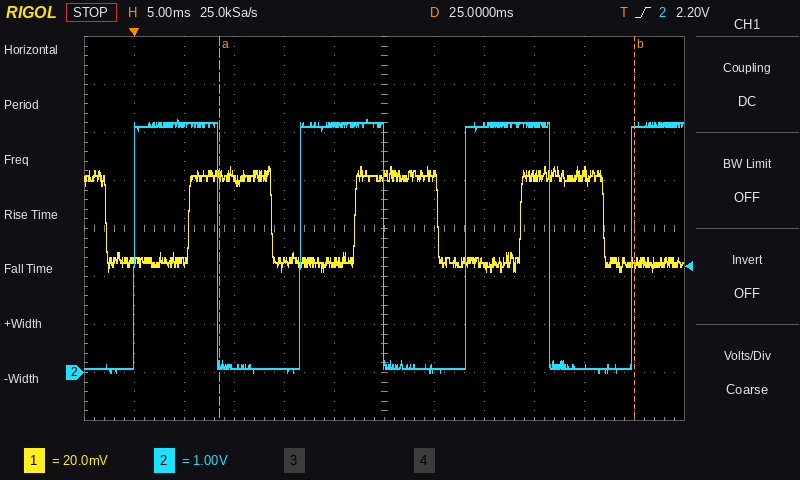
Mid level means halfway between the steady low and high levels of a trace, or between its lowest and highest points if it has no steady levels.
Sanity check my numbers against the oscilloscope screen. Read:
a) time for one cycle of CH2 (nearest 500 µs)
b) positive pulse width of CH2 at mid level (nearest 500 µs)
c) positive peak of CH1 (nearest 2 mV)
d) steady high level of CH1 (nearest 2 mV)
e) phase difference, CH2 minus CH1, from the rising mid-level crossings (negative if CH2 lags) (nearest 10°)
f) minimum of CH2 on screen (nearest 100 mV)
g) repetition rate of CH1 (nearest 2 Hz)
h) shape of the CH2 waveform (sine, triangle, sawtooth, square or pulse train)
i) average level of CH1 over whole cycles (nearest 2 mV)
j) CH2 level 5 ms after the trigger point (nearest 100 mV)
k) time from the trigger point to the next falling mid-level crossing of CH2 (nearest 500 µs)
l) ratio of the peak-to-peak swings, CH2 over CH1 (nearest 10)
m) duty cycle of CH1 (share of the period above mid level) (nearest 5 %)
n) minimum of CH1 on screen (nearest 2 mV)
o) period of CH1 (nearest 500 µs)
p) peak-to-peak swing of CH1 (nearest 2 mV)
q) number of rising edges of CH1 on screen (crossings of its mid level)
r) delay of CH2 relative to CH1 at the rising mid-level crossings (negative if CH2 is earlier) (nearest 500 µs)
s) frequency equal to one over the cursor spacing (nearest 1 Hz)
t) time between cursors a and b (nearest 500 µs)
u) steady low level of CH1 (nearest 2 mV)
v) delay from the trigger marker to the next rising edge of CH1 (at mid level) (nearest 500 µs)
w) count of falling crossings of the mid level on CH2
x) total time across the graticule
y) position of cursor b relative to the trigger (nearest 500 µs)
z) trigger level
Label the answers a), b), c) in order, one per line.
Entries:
a) 16.5 ms
b) 8.5 ms
c) 86 mV
d) 82 mV
e) +120°
f) 0.0 V
g) 60 Hz
h) square
i) 64 mV
j) 5.2 V
k) 8.5 ms
l) 120
m) 50 %
n) 42 mV
o) 16.5 ms
p) 44 mV
q) 3
r) -5.5 ms
s) 24 Hz
t) 41.5 ms
u) 46 mV
v) 5.5 ms
w) 3
x) 60 ms
y) +50.0 ms
z) 2.20 V
